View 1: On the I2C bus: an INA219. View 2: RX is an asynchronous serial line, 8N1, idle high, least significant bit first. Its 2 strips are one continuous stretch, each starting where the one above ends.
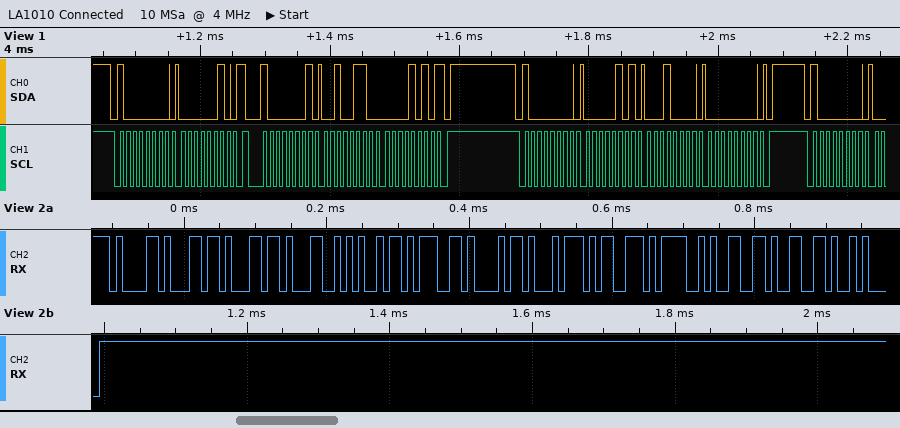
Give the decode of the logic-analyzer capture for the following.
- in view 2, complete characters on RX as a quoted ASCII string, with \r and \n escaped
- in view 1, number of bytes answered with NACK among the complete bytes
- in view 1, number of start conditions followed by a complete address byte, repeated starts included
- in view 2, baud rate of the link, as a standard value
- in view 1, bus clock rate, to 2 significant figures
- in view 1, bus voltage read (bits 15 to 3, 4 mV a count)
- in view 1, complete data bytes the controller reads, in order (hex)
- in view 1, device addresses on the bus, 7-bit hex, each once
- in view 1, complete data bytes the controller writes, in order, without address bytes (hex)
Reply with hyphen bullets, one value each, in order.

- "allLightsOff\n"
- 1
- 4
- 115200 baud
- 100 kHz
- 4.868 V
- 26 0A
- 0x40
- 02 05 10 00
